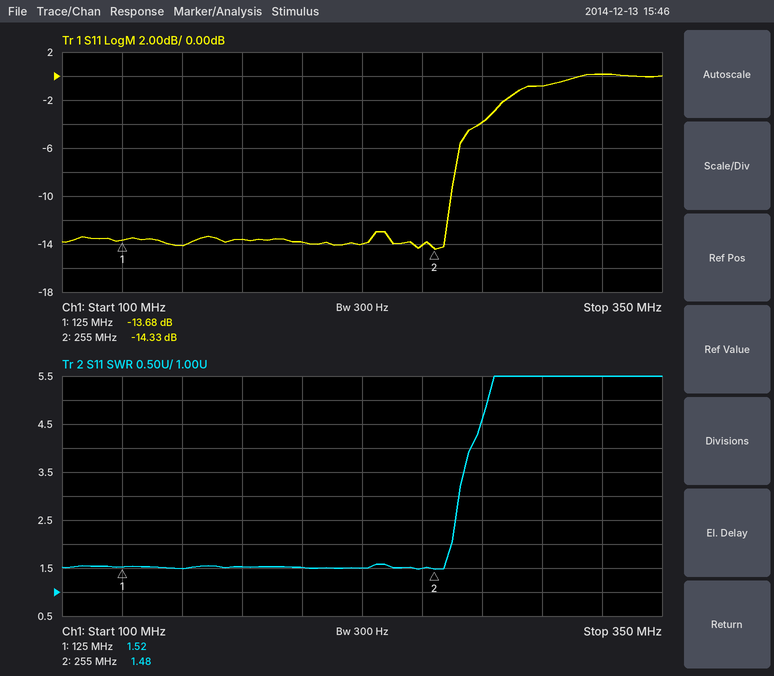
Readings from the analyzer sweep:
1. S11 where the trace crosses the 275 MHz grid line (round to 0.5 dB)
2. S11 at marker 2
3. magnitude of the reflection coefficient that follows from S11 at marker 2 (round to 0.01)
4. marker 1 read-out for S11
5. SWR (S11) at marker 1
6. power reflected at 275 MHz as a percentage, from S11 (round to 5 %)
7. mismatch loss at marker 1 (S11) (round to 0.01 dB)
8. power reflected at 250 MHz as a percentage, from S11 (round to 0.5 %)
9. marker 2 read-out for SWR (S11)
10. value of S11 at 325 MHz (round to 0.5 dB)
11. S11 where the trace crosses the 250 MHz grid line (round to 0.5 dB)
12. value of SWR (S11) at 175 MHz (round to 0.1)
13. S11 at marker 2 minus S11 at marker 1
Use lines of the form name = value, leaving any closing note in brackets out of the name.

S11 where the trace crosses the 275 MHz grid line = -4.0 dB
S11 at marker 2 = -14.33 dB
magnitude of the reflection coefficient that follows from S11 at marker 2 = 0.19
marker 1 read-out for S11 = -13.68 dB
SWR (S11) at marker 1 = 1.52
power reflected at 275 MHz as a percentage, from S11 = 40 %
mismatch loss at marker 1 (S11) = 0.19 dB
power reflected at 250 MHz as a percentage, from S11 = 4.0 %
marker 2 read-out for SWR = 1.48
value of S11 at 325 MHz = 0.0 dB
S11 where the trace crosses the 250 MHz grid line = -14.0 dB
value of SWR (S11) at 175 MHz = 1.5
S11 at marker 2 minus S11 at marker 1 = -0.65 dB
